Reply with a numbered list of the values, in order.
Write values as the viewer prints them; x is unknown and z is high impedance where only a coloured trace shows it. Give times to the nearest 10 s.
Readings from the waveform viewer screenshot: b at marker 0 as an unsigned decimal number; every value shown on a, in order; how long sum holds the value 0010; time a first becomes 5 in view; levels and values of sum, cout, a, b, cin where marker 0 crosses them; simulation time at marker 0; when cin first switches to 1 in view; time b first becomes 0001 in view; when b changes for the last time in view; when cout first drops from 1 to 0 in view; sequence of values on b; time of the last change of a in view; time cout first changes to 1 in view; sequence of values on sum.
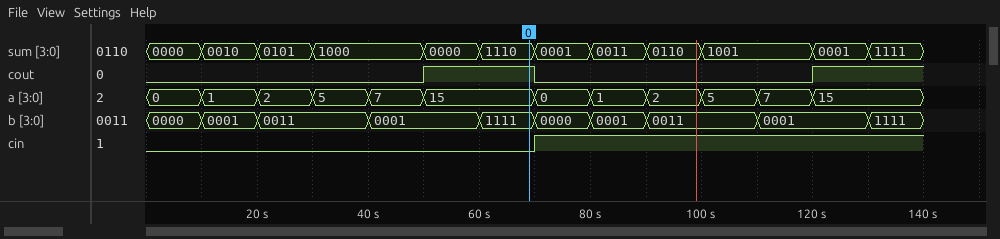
1. 15
2. 0, 1, 2, 5, 7, 15, 0, 1, 2, 5, 7, 15
3. 10 s
4. 30 s
5. sum=1110, cout=1, a=15, b=1111, cin=0
6. 70 s
7. 70 s
8. 10 s
9. 130 s
10. 70 s
11. 0000, 0001, 0011, 0001, 1111, 0000, 0001, 0011, 0001, 1111
12. 120 s
13. 50 s
14. 0000, 0010, 0101, 1000, 0000, 1110, 0001, 0011, 0110, 1001, 0001, 1111
